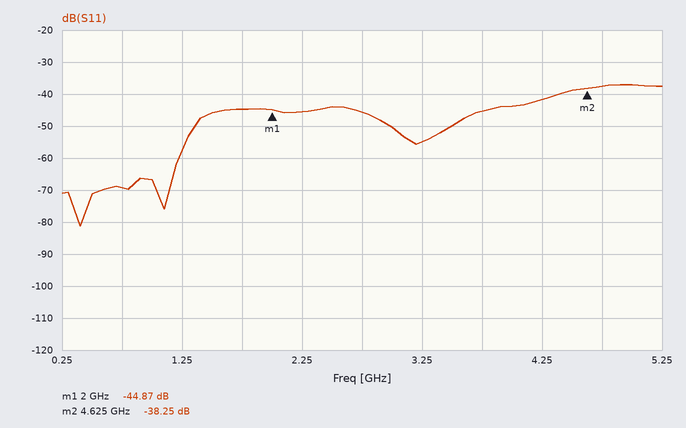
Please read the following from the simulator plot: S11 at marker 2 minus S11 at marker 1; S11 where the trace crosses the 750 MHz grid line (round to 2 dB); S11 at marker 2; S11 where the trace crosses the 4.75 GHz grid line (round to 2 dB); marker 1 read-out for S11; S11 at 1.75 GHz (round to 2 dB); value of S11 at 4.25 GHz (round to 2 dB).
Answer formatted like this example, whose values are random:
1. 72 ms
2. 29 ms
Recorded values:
1. 6.62 dB
2. -70 dB
3. -38.25 dB
4. -38 dB
5. -44.87 dB
6. -44 dB
7. -42 dB
